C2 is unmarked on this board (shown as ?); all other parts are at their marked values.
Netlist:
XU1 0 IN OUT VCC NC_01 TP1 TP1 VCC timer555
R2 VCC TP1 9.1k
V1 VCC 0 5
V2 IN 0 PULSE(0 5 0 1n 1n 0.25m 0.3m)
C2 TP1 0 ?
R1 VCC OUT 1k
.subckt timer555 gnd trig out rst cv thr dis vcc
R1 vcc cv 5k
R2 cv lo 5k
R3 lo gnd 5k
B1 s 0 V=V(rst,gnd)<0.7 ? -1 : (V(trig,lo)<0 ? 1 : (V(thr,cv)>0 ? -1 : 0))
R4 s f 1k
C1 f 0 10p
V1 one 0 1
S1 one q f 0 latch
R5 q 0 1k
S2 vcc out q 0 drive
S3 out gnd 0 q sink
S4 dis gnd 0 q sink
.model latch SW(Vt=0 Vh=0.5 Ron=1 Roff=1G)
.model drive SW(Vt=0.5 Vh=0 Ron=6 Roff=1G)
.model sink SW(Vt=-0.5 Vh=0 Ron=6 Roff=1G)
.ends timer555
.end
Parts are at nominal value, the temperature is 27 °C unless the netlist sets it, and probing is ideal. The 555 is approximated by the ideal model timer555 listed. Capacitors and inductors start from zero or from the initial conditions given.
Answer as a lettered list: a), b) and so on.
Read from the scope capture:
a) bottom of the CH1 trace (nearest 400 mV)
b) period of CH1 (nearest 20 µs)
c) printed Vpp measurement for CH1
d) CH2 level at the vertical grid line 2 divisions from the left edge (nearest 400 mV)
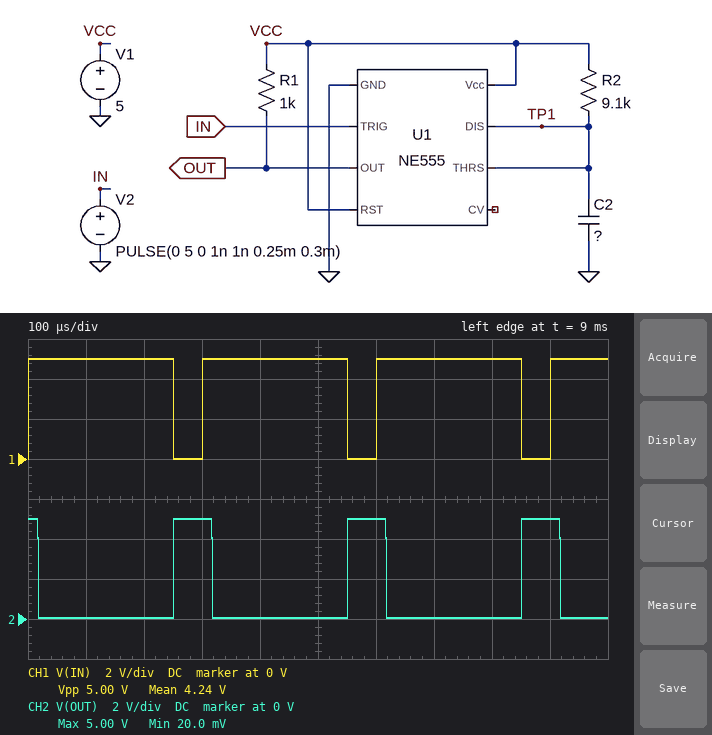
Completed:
a) 0 V
b) 300 µs
c) 5.00 V
d) 0 V
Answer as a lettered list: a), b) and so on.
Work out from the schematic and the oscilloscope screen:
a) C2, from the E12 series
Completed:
a) 6.8 nF
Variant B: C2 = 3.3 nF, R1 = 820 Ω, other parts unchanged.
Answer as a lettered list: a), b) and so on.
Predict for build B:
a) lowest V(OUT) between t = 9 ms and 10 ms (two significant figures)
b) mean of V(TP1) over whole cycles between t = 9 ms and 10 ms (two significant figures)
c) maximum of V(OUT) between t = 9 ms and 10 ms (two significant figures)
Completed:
a) 36 mV
b) 430 mV
c) 5.0 V
